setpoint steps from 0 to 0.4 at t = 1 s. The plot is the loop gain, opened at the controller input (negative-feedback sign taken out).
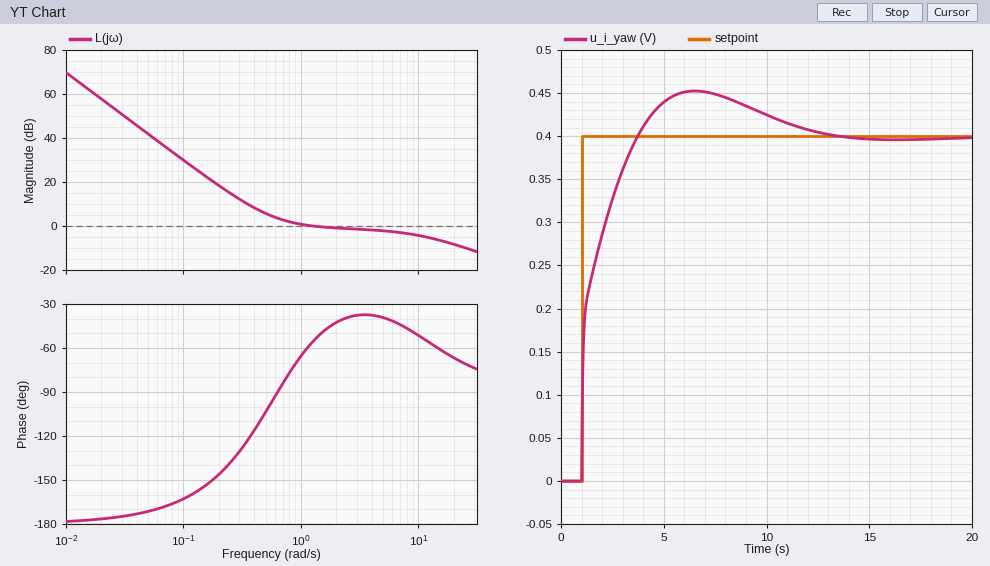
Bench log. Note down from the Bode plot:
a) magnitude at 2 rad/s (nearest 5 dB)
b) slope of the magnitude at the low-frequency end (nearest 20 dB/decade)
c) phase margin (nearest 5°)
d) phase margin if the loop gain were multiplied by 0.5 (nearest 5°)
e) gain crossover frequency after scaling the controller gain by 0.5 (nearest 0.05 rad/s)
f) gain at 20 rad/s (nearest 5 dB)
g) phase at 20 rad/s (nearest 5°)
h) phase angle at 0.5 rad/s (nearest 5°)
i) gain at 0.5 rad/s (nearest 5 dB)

0 dB
-40 dB/decade
125°
75°
0.50 rad/s
-10 dB
-65°
-105°
5 dB
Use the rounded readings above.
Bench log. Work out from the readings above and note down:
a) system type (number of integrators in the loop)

2
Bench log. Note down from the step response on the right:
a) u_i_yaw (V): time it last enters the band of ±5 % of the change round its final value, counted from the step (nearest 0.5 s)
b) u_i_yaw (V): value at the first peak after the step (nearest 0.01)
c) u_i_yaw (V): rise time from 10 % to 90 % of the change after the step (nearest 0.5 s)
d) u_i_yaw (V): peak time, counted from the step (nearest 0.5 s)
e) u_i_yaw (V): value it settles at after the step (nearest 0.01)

9.5 s
0.45
2.0 s
5.5 s
0.40
